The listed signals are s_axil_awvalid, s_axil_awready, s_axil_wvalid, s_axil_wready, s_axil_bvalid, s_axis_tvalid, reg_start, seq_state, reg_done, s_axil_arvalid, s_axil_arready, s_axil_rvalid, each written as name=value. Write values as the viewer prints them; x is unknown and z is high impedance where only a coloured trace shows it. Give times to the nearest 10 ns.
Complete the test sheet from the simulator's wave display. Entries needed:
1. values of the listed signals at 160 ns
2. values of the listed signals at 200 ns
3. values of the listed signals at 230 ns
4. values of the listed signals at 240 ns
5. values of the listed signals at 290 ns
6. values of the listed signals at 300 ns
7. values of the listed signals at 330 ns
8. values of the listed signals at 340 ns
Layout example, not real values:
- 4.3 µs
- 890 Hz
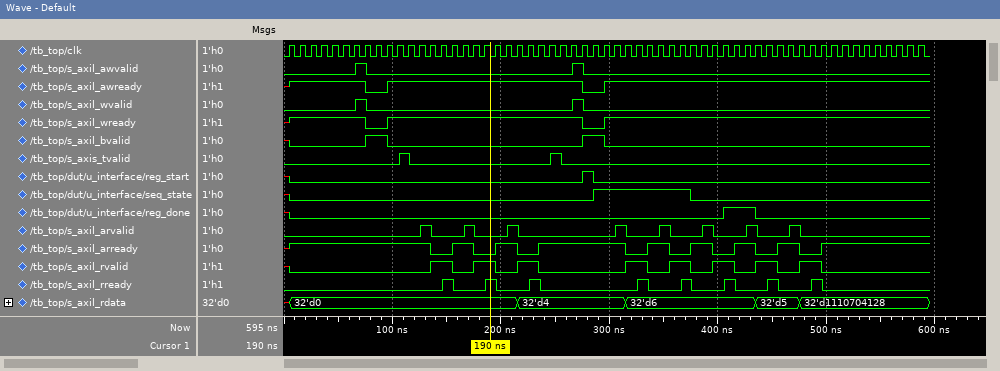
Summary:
- s_axil_awvalid=0, s_axil_awready=1, s_axil_wvalid=0, s_axil_wready=1, s_axil_bvalid=0, s_axis_tvalid=0, reg_start=0, seq_state=0, reg_done=0, s_axil_arvalid=0, s_axil_arready=1, s_axil_rvalid=0
- s_axil_awvalid=0, s_axil_awready=1, s_axil_wvalid=0, s_axil_wready=1, s_axil_bvalid=0, s_axis_tvalid=0, reg_start=0, seq_state=0, reg_done=0, s_axil_arvalid=0, s_axil_arready=1, s_axil_rvalid=0
- s_axil_awvalid=0, s_axil_awready=1, s_axil_wvalid=0, s_axil_wready=1, s_axil_bvalid=0, s_axis_tvalid=0, reg_start=0, seq_state=0, reg_done=0, s_axil_arvalid=0, s_axil_arready=0, s_axil_rvalid=1
- s_axil_awvalid=0, s_axil_awready=1, s_axil_wvalid=0, s_axil_wready=1, s_axil_bvalid=0, s_axis_tvalid=0, reg_start=0, seq_state=0, reg_done=0, s_axil_arvalid=0, s_axil_arready=1, s_axil_rvalid=0
- s_axil_awvalid=0, s_axil_awready=0, s_axil_wvalid=0, s_axil_wready=0, s_axil_bvalid=1, s_axis_tvalid=0, reg_start=0, seq_state=1, reg_done=0, s_axil_arvalid=0, s_axil_arready=1, s_axil_rvalid=0
- s_axil_awvalid=0, s_axil_awready=1, s_axil_wvalid=0, s_axil_wready=1, s_axil_bvalid=0, s_axis_tvalid=0, reg_start=0, seq_state=1, reg_done=0, s_axil_arvalid=0, s_axil_arready=1, s_axil_rvalid=0
- s_axil_awvalid=0, s_axil_awready=1, s_axil_wvalid=0, s_axil_wready=1, s_axil_bvalid=0, s_axis_tvalid=0, reg_start=0, seq_state=1, reg_done=0, s_axil_arvalid=0, s_axil_arready=0, s_axil_rvalid=1
- s_axil_awvalid=0, s_axil_awready=1, s_axil_wvalid=0, s_axil_wready=1, s_axil_bvalid=0, s_axis_tvalid=0, reg_start=0, seq_state=1, reg_done=0, s_axil_arvalid=0, s_axil_arready=1, s_axil_rvalid=0
